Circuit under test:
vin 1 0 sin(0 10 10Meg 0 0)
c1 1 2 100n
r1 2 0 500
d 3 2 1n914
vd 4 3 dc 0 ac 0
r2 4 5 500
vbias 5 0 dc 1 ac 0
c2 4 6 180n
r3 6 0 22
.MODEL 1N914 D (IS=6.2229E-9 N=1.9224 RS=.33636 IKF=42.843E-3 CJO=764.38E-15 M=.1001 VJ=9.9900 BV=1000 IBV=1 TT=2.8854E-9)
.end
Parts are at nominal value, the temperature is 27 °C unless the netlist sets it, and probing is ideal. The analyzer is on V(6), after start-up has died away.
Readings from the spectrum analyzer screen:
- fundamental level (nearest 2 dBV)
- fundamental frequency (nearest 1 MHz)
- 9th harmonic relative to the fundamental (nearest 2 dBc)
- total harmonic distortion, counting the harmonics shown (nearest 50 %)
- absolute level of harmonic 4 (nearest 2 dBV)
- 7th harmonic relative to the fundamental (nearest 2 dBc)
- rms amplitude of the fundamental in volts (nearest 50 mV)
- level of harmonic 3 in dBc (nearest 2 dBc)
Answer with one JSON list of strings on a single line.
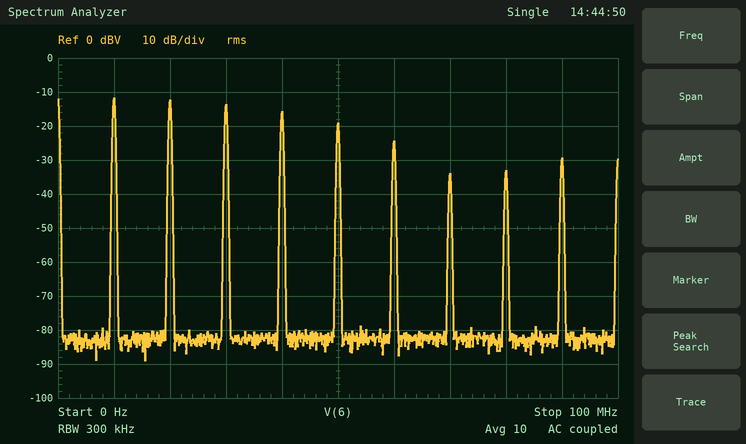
["-12 dBV", "10 MHz", "-18 dBc", "150 %", "-16 dBV", "-22 dBc", "250 mV", "-2 dBc"]
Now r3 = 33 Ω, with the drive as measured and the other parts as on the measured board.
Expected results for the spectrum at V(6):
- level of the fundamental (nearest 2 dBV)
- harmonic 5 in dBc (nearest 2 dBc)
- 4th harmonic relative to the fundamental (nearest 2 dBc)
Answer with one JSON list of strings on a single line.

["-8 dBV", "-10 dBc", "-6 dBc"]
